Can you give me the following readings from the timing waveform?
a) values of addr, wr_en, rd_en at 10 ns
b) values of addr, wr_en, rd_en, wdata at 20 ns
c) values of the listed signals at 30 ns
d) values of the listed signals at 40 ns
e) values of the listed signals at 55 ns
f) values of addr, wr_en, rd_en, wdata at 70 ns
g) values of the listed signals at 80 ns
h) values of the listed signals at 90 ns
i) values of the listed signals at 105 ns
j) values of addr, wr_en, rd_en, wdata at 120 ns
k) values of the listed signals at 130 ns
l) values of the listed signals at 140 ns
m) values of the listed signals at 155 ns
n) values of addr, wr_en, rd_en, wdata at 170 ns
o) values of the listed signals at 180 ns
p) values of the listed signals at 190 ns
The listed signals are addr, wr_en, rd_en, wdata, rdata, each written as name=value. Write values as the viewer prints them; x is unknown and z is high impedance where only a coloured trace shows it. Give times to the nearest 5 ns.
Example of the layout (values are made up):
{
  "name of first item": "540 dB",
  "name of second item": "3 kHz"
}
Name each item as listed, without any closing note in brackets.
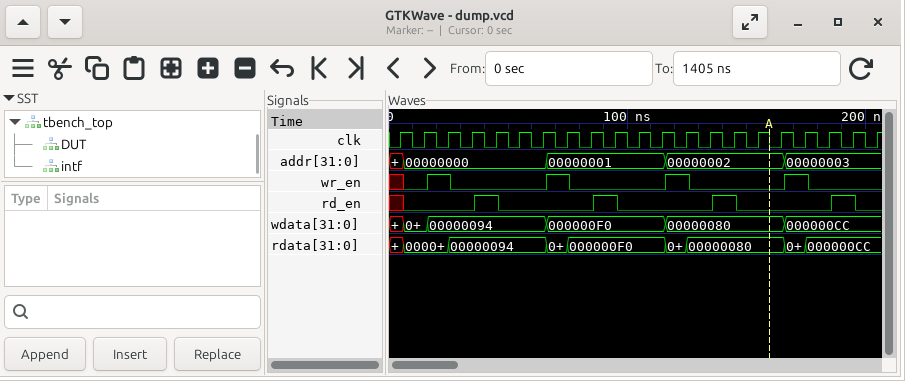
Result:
{
  "values of addr, wr_en, rd_en at 10 ns": "addr=00000000, wr_en=0, rd_en=0",
  "values of addr, wr_en, rd_en, wdata at 20 ns": "addr=00000000, wr_en=1, rd_en=0, wdata=00000094",
  "values of the listed signals at 30 ns": "addr=00000000, wr_en=0, rd_en=0, wdata=00000094, rdata=00000094",
  "values of the listed signals at 40 ns": "addr=00000000, wr_en=0, rd_en=1, wdata=00000094, rdata=00000094",
  "values of the listed signals at 55 ns": "addr=00000000, wr_en=0, rd_en=0, wdata=00000094, rdata=00000094",
  "values of addr, wr_en, rd_en, wdata at 70 ns": "addr=00000001, wr_en=1, rd_en=0, wdata=000000F0",
  "values of the listed signals at 80 ns": "addr=00000001, wr_en=0, rd_en=0, wdata=000000F0, rdata=000000F0",
  "values of the listed signals at 90 ns": "addr=00000001, wr_en=0, rd_en=1, wdata=000000F0, rdata=000000F0",
  "values of the listed signals at 105 ns": "addr=00000001, wr_en=0, rd_en=0, wdata=000000F0, rdata=000000F0",
  "values of addr, wr_en, rd_en, wdata at 120 ns": "addr=00000002, wr_en=1, rd_en=0, wdata=00000080",
  "values of the listed signals at 130 ns": "addr=00000002, wr_en=0, rd_en=0, wdata=00000080, rdata=00000080",
  "values of the listed signals at 140 ns": "addr=00000002, wr_en=0, rd_en=1, wdata=00000080, rdata=00000080",
  "values of the listed signals at 155 ns": "addr=00000002, wr_en=0, rd_en=0, wdata=00000080, rdata=00000080",
  "values of addr, wr_en, rd_en, wdata at 170 ns": "addr=00000003, wr_en=1, rd_en=0, wdata=000000CC",
  "values of the listed signals at 180 ns": "addr=00000003, wr_en=0, rd_en=0, wdata=000000CC, rdata=000000CC",
  "values of the listed signals at 190 ns": "addr=00000003, wr_en=0, rd_en=1, wdata=000000CC, rdata=000000CC"
}
